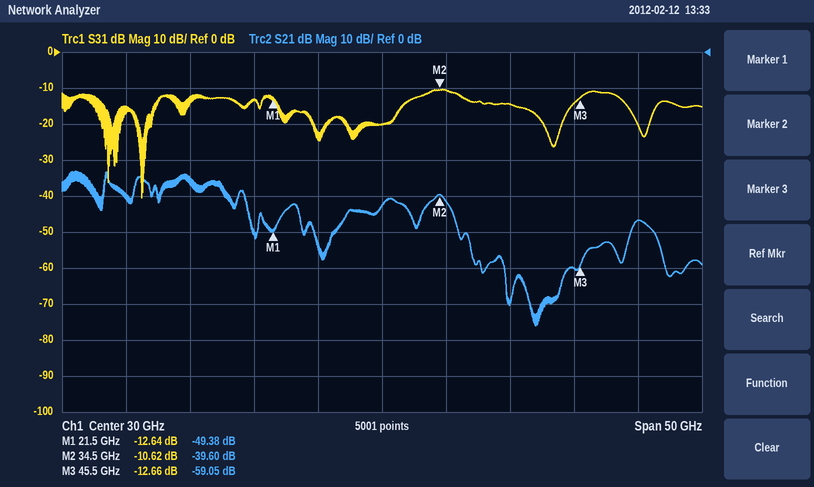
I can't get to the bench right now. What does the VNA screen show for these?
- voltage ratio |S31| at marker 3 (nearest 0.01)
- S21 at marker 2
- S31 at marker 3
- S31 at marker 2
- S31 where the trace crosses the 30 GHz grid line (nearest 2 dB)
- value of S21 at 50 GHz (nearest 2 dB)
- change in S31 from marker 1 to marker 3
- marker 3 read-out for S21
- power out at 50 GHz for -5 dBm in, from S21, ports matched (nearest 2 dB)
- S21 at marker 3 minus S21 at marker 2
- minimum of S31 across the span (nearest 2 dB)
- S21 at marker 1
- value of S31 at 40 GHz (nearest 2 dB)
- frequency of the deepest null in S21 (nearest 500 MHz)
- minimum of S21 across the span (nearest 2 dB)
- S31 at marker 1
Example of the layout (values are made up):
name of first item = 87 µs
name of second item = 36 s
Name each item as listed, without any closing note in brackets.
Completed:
voltage ratio |S31| at marker 3 = 0.23
S21 at marker 2 = -39.60 dB
S31 at marker 3 = -12.66 dB
S31 at marker 2 = -10.62 dB
S31 where the trace crosses the 30 GHz grid line = -20 dB
value of S21 at 50 GHz = -46 dB
change in S31 from marker 1 to marker 3 = -0.02 dB
marker 3 read-out for S21 = -59.05 dB
power out at 50 GHz for -5 dBm in, from S21, ports matched = -52 dBm
S21 at marker 3 minus S21 at marker 2 = -19.45 dB
minimum of S31 across the span = -40 dB
S21 at marker 1 = -49.38 dB
value of S31 at 40 GHz = -14 dB
frequency of the deepest null in S21 = 42.0 GHz
minimum of S21 across the span = -76 dB
S31 at marker 1 = -12.64 dB
